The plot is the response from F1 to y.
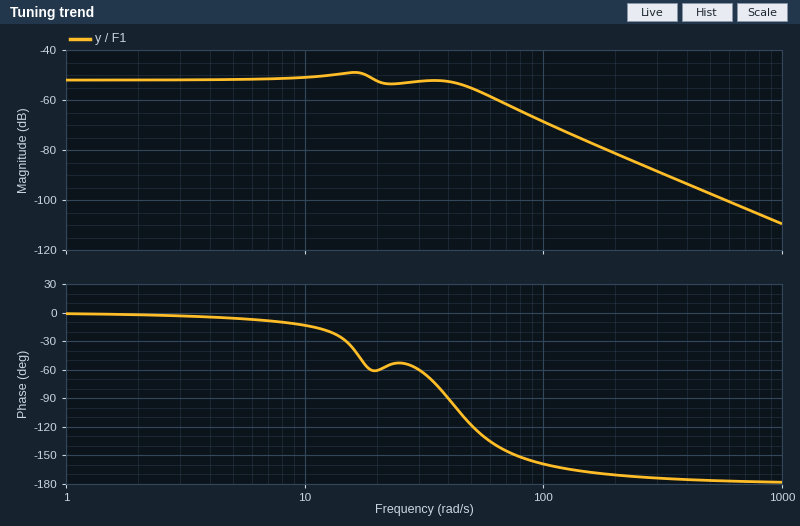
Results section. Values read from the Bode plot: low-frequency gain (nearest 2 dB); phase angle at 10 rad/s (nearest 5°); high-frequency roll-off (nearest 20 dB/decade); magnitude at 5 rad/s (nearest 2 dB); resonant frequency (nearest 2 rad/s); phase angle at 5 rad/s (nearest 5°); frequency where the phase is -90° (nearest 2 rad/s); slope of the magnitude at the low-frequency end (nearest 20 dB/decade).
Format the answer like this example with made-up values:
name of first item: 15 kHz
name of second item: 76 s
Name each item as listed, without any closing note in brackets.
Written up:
low-frequency gain: -52 dB
phase angle at 10 rad/s: -15°
high-frequency roll-off: -40 dB/decade
magnitude at 5 rad/s: -52 dB
resonant frequency: 16 rad/s
phase angle at 5 rad/s: -5°
frequency where the phase is -90°: 40 rad/s
slope of the magnitude at the low-frequency end: 0 dB/decade
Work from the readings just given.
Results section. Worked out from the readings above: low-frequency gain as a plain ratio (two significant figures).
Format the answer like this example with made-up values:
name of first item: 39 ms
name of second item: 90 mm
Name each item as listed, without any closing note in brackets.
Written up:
low-frequency gain as a plain ratio: 0.0025
